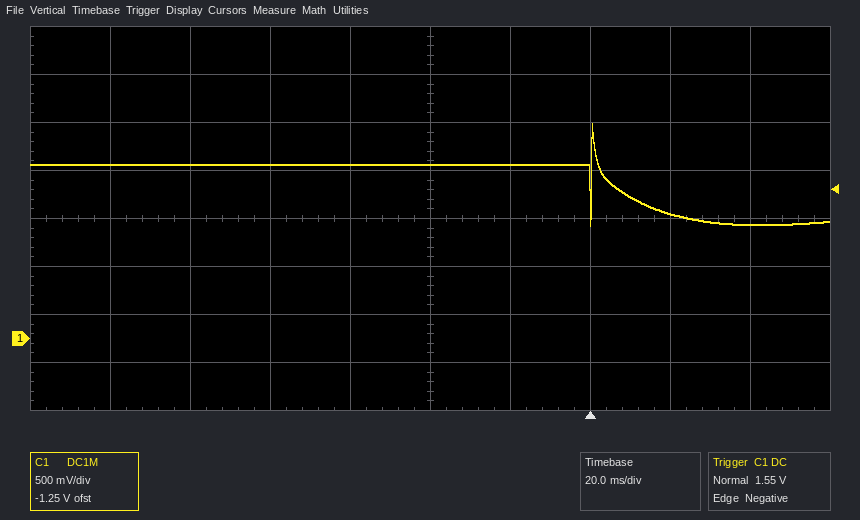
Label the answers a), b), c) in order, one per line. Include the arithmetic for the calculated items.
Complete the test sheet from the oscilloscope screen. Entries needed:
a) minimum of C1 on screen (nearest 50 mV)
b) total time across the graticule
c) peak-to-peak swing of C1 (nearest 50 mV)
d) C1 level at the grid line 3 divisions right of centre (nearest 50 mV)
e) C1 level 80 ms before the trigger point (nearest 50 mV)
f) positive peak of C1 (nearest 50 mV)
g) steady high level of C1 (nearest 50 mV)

a) 1.20 V
b) 200 ms
c) 2.25 V − (1.20 V) = 1.05 V
d) 1.30 V
e) 1.80 V
f) 2.25 V
g) 1.80 V
